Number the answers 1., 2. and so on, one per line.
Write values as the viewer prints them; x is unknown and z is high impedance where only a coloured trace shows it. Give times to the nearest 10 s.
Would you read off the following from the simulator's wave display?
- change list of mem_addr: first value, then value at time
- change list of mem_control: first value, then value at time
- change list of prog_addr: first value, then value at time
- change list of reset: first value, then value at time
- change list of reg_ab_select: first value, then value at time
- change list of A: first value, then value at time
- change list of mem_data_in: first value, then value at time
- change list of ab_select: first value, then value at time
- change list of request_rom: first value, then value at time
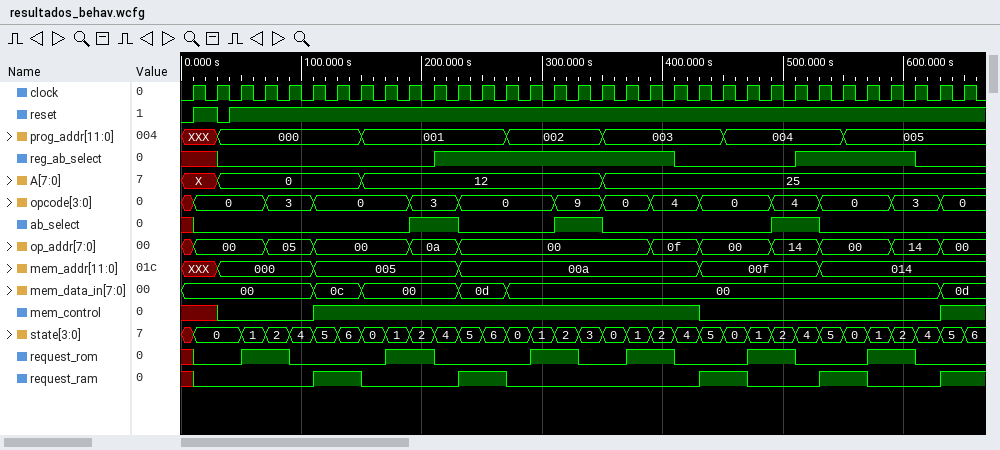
1. XXX, 000 at 30 s, 005 at 110 s, 00a at 230 s, 00f at 430 s, 014 at 530 s
2. x, 0 at 30 s, 1 at 110 s, 0 at 430 s, 1 at 630 s
3. XXX, 000 at 30 s, 001 at 150 s, 002 at 270 s, 003 at 350 s, 004 at 450 s, 005 at 550 s
4. 0, 1 at 10 s, 0 at 30 s, 1 at 40 s
5. x, 0 at 30 s, 1 at 210 s, 0 at 410 s, 1 at 510 s, 0 at 610 s
6. X, 0 at 30 s, 12 at 150 s, 25 at 350 s
7. 00, 0c at 110 s, 00 at 150 s, 0d at 230 s, 00 at 270 s, 0d at 630 s
8. x, 0 at 10 s, 1 at 190 s, 0 at 230 s, 1 at 310 s, 0 at 350 s, 1 at 490 s, 0 at 530 s
9. x, 0 at 10 s, 1 at 50 s, 0 at 90 s, 1 at 170 s, 0 at 210 s, 1 at 290 s, 0 at 330 s, 1 at 370 s, 0 at 410 s, 1 at 470 s, 0 at 510 s, 1 at 570 s, 0 at 610 s
